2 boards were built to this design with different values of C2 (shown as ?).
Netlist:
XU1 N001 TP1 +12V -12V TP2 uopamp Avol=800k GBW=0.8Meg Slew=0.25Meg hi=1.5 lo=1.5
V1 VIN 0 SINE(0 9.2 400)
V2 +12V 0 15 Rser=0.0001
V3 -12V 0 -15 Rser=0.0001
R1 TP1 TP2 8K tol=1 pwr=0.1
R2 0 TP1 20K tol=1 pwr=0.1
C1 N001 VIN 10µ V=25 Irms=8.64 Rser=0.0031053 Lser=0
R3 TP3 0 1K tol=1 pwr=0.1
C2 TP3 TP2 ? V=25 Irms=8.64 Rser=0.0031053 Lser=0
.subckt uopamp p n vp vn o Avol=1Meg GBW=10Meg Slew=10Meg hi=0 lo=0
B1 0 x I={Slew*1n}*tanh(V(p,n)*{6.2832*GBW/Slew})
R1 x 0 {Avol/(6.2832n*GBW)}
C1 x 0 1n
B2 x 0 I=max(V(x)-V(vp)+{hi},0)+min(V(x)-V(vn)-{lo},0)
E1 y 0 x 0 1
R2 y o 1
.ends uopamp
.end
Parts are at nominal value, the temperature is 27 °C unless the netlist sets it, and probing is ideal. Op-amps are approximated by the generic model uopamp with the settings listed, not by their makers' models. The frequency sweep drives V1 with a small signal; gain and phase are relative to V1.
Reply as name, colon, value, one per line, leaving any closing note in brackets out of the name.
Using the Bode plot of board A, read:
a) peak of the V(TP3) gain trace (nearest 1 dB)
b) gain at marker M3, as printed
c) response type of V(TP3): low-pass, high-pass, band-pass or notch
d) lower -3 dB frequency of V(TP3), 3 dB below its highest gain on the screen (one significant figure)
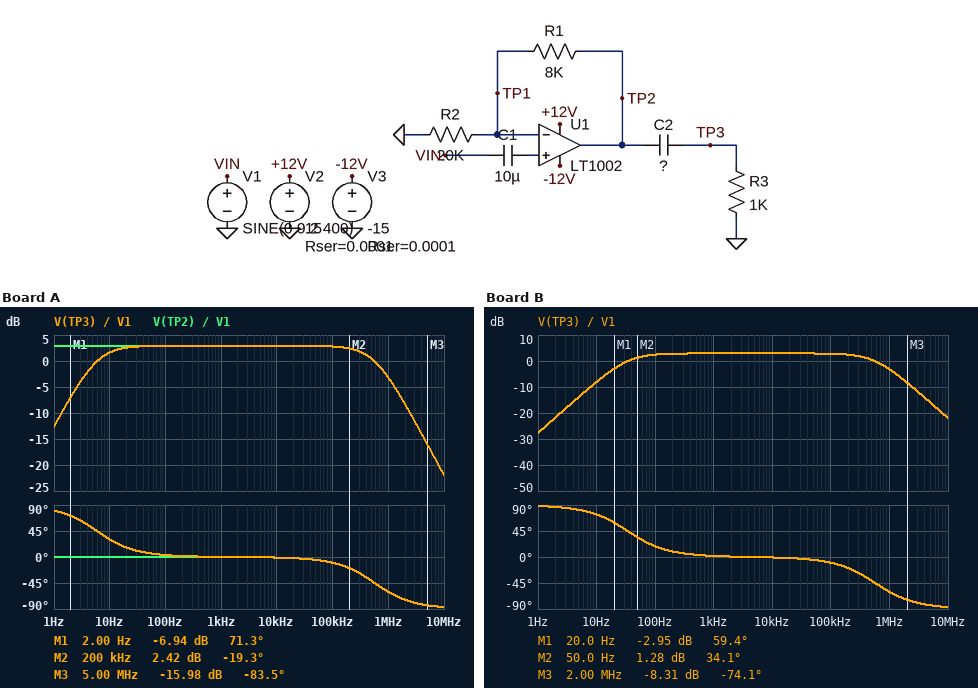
peak of the V(TP3) gain trace: 3 dB
gain at marker M3, as printed: -15.98 dB
response type of V(TP3): low-pass, high-pass, band-pass or notch: band-pass
lower -3 dB frequency of V(TP3), 3 dB below its highest gain on the screen: 6 Hz
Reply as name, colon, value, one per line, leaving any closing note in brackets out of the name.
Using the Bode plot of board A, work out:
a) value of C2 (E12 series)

value of C2: 27 µF
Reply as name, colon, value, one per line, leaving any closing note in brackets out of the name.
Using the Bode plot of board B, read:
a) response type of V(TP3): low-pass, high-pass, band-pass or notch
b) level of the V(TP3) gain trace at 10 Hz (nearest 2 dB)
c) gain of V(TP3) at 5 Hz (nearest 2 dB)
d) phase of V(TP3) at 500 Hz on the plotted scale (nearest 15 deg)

response type of V(TP3): low-pass, high-pass, band-pass or notch: band-pass
level of the V(TP3) gain trace at 10 Hz: -8 dB
gain of V(TP3) at 5 Hz: -14 dB
phase of V(TP3) at 500 Hz on the plotted scale: 0 deg
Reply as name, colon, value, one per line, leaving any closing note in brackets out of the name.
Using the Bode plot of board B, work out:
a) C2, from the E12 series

C2, from the E12 series: 4.7 µF
